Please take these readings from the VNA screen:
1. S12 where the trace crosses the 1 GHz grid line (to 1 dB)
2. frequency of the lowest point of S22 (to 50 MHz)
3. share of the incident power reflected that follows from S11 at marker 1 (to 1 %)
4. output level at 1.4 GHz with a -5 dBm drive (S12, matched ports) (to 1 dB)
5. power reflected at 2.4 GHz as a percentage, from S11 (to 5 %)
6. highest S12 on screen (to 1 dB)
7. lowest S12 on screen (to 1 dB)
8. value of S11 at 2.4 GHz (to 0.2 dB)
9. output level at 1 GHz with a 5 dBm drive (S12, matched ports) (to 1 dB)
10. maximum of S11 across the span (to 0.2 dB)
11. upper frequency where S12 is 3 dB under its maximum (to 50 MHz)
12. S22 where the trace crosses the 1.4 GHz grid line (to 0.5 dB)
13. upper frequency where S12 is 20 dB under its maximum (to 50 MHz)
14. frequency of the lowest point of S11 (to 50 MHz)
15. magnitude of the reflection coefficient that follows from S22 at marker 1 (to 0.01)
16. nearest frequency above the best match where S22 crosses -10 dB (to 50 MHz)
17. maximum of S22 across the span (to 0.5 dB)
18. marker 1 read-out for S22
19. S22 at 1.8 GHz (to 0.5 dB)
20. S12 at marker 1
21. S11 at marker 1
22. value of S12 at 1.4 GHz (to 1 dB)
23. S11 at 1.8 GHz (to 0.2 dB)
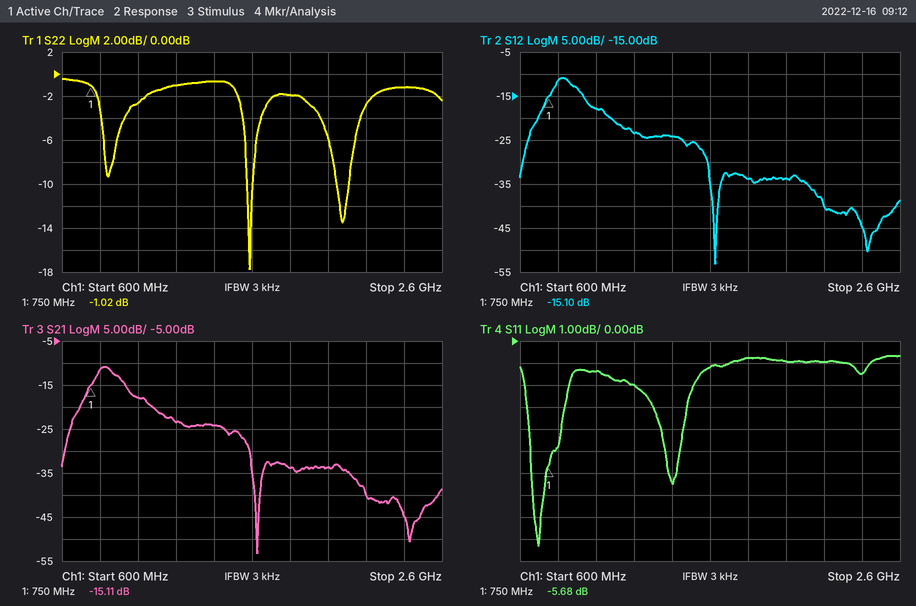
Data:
-18 dB
1.60 GHz
27 %
-29 dBm
70 %
-11 dB
-53 dB
-1.4 dB
-13 dBm
-0.6 dB
900 MHz
-0.5 dB
1.60 GHz
700 MHz
0.89
1.60 GHz
-0.5 dB
-1.02 dB
-2.0 dB
-15.10 dB
-5.68 dB
-24 dB
-0.8 dB
